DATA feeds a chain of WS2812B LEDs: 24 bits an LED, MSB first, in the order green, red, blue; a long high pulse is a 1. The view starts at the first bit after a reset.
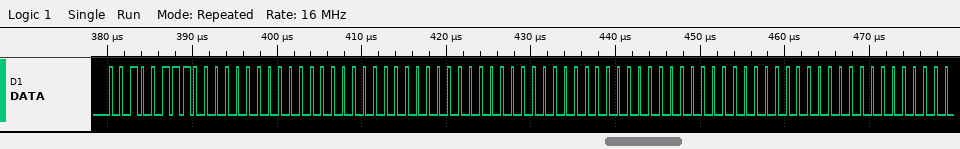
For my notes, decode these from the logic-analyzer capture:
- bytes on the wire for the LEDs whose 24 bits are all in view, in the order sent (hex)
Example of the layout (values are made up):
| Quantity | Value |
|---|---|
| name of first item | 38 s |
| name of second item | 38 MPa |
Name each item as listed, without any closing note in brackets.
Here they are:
| Quantity | Value |
|---|---|
| bytes on the wire for the LEDs whose 24 bits are all in view, in the order sent | 27 00 00 00 00 00 00 00 00 |
